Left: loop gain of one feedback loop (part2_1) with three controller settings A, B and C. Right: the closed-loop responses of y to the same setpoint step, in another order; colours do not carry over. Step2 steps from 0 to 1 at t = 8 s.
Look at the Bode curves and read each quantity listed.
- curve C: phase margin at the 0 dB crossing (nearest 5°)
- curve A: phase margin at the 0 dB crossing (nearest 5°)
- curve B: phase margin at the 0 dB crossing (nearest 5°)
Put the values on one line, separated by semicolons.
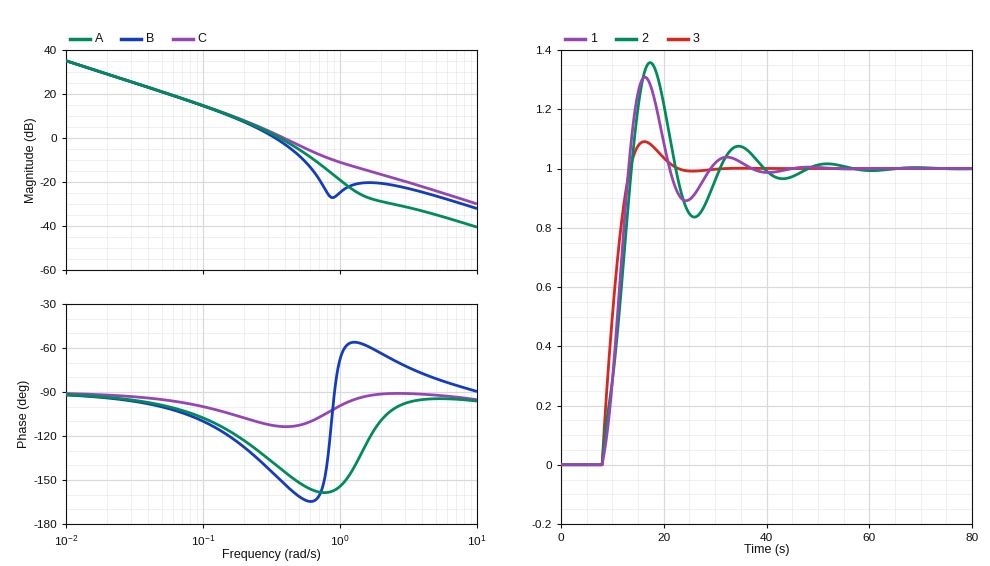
65°; 40°; 35°
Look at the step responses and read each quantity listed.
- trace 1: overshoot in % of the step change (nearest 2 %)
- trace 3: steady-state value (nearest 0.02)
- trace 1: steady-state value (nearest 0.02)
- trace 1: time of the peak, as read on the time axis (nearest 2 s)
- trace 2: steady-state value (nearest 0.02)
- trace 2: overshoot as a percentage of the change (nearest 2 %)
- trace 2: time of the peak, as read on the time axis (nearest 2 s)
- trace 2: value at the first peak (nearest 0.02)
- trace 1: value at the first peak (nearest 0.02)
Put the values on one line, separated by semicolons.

30 %; 1.00; 1.00; 16 s; 1.00; 36 %; 18 s; 1.36; 1.30
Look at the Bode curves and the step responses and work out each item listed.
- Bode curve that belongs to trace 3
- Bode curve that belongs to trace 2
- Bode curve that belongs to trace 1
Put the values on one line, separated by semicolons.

C; B; A
